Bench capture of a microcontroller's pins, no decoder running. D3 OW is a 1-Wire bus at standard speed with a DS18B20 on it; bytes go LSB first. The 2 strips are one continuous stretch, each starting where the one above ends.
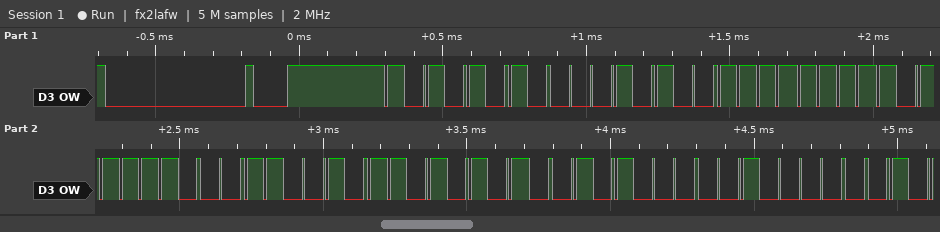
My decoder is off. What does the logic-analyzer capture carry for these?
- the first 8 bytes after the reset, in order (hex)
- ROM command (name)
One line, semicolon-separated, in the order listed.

55 28 FF 7D 4C AB 14 04; Match ROM
